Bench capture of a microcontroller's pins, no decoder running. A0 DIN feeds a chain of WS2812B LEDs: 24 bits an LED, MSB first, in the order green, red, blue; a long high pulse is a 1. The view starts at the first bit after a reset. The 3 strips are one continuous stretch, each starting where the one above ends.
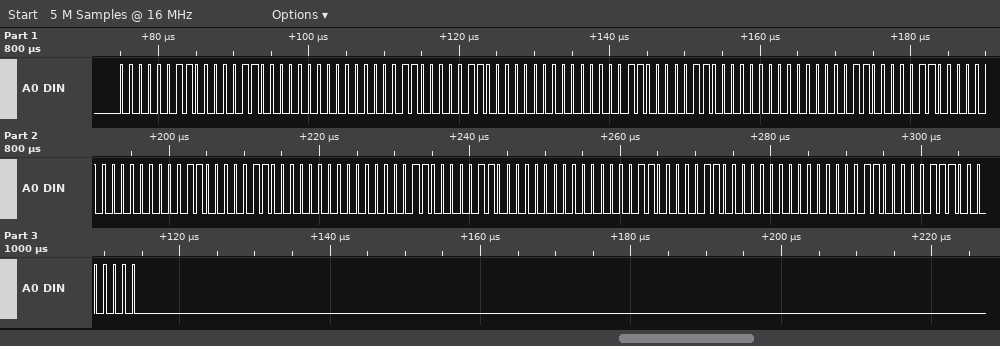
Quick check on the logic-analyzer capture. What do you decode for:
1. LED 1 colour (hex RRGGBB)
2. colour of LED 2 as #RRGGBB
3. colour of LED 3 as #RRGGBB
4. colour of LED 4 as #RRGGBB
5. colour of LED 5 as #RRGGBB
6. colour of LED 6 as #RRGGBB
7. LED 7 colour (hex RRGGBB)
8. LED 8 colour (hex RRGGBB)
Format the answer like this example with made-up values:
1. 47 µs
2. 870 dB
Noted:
1. #060300
2. #060300
3. #060300
4. #060300
5. #060300
6. #060300
7. #060300
8. #070300
